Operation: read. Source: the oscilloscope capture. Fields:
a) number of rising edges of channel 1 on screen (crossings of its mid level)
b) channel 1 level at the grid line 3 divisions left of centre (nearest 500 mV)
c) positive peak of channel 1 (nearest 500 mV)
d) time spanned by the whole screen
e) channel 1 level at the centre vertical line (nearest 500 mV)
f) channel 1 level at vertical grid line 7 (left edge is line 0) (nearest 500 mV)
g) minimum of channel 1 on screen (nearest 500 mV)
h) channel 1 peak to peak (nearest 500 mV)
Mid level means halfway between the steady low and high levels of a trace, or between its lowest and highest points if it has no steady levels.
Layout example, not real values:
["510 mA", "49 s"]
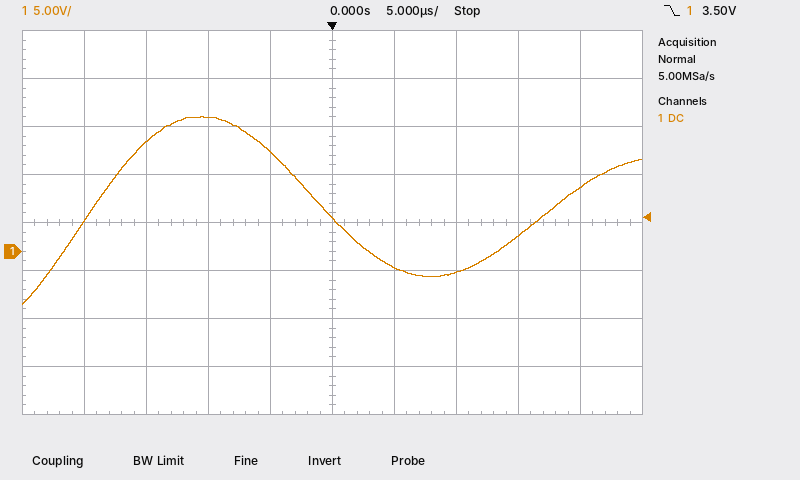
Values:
["2", "11.5 V", "14.0 V", "50 µs", "3.5 V", "-2.0 V", "-5.5 V", "19.5 V"]
